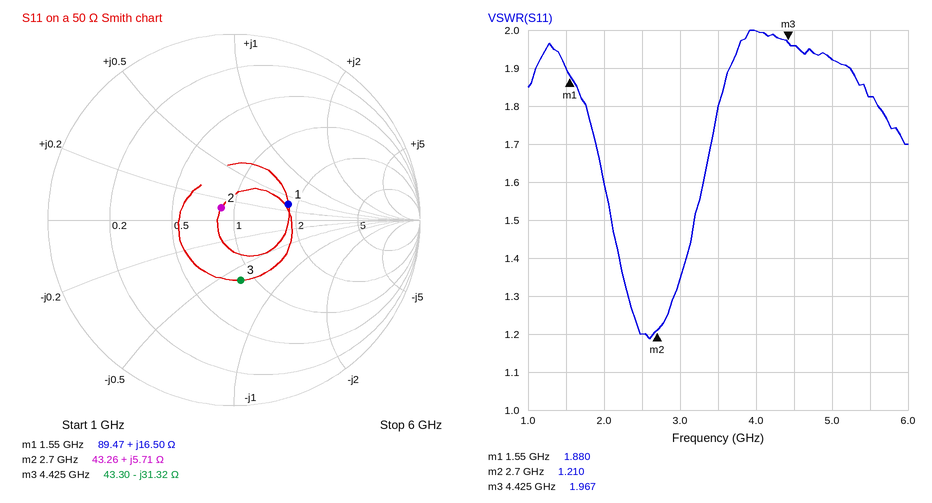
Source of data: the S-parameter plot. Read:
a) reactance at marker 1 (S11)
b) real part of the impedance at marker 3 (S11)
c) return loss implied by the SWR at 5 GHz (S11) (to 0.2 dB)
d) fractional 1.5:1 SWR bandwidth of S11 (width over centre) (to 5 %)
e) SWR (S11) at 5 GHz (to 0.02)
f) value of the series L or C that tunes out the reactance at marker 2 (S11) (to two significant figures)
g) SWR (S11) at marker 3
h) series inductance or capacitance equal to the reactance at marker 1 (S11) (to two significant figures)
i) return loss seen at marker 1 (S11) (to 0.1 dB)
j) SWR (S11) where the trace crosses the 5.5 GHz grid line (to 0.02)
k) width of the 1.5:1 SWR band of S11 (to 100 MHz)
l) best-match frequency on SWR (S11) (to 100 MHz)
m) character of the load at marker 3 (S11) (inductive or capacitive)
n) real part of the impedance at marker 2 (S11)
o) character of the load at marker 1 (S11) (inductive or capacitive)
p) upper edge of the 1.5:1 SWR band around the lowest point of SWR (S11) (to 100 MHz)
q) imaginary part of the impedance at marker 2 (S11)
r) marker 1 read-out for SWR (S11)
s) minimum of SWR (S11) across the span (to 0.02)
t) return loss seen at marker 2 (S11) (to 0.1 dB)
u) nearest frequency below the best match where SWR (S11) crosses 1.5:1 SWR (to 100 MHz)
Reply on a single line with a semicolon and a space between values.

+16.50 Ω; 43.30 Ω; 10.0 dB; 40 %; 1.92; 10 pF; 1.967; 1.7 nH; 10.3 dB; 1.82; 1.1 GHz; 2.6 GHz; capacitive; 43.26 Ω; inductive; 3.2 GHz; +5.71 Ω; 1.880; 1.18; 20.5 dB; 2.1 GHz
